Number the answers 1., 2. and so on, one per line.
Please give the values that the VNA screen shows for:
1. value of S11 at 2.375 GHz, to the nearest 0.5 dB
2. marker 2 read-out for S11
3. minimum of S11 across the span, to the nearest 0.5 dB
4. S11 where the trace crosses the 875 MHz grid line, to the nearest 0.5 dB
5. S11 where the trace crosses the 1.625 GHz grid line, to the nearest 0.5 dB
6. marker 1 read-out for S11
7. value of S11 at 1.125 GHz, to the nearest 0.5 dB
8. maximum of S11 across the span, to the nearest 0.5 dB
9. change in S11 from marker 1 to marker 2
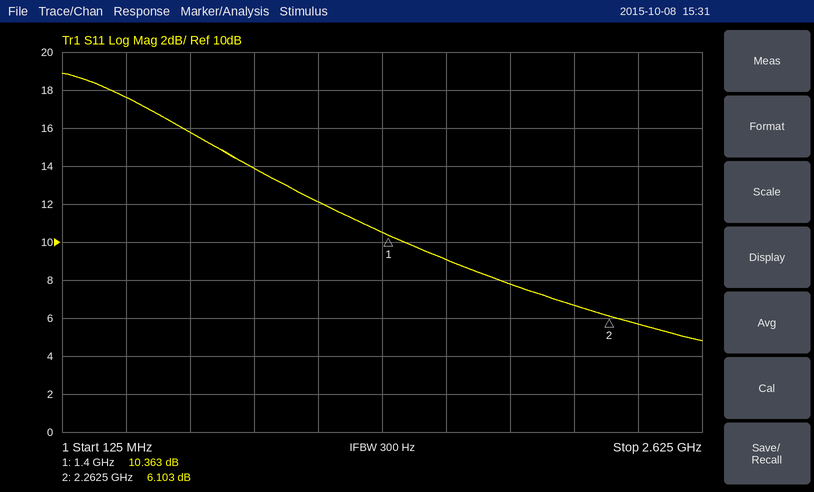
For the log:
1. 5.5 dB
2. 6.103 dB
3. 5.0 dB
4. 14.0 dB
5. 9.0 dB
6. 10.363 dB
7. 12.0 dB
8. 19.0 dB
9. -4.260 dB
